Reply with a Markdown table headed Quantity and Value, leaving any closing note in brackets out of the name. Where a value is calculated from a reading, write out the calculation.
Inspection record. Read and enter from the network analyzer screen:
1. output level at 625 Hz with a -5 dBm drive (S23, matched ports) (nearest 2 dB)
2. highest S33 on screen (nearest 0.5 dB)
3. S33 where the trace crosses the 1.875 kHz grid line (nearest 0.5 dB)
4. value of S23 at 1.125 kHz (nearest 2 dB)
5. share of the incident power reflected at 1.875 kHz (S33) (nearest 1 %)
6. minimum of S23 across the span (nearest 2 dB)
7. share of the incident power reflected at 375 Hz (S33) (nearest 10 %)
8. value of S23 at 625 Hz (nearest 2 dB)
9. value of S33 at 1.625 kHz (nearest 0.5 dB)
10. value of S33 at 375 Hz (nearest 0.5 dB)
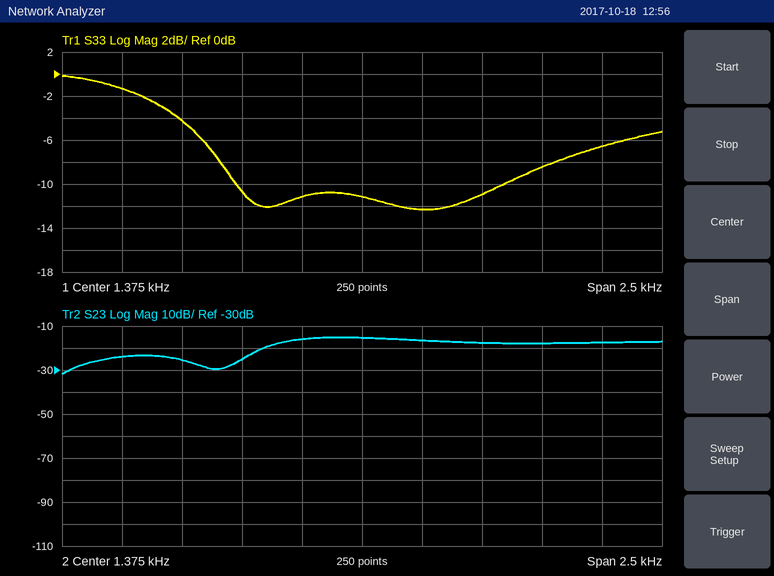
| Quantity | Value |
|---|---|
| output level at 625 Hz with a -5 dBm drive (S23, matched ports) | -5 dBm + (-26 dB) = -30 dBm |
| highest S33 on screen | 0.0 dB |
| S33 where the trace crosses the 1.875 kHz grid line | -11.0 dB |
| value of S23 at 1.125 kHz | -16 dB |
| share of the incident power reflected at 1.875 kHz (S33) | 10^(-11/10) ≈ 8 % |
| minimum of S23 across the span | -32 dB |
| share of the incident power reflected at 375 Hz (S33) | 10^(-1.5/10) ≈ 70.8 %, so 70 % to the nearest 10 % |
| value of S23 at 625 Hz | -26 dB |
| value of S33 at 1.625 kHz | -12.5 dB |
| value of S33 at 375 Hz | -1.5 dB |
